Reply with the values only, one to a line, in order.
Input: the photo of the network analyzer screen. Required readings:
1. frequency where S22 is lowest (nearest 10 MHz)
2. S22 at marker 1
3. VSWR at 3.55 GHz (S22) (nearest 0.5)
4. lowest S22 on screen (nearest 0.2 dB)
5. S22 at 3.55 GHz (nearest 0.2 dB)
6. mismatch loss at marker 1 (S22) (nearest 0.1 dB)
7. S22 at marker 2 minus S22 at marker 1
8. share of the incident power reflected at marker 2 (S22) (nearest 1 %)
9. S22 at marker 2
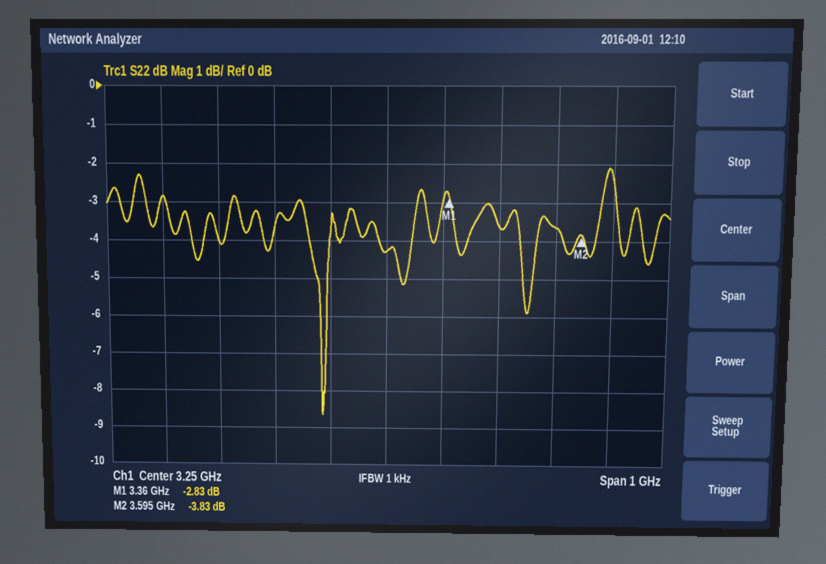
3.14 GHz
-2.83 dB
5.0
-8.6 dB
-3.6 dB
3.2 dB
-1.00 dB
41 %
-3.83 dB
